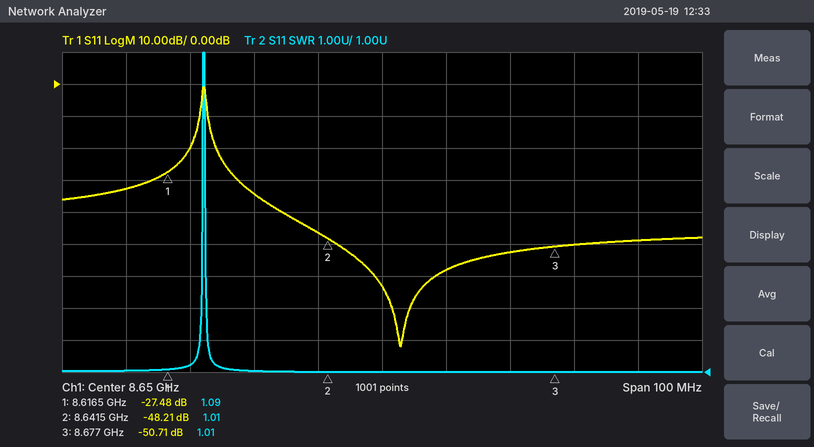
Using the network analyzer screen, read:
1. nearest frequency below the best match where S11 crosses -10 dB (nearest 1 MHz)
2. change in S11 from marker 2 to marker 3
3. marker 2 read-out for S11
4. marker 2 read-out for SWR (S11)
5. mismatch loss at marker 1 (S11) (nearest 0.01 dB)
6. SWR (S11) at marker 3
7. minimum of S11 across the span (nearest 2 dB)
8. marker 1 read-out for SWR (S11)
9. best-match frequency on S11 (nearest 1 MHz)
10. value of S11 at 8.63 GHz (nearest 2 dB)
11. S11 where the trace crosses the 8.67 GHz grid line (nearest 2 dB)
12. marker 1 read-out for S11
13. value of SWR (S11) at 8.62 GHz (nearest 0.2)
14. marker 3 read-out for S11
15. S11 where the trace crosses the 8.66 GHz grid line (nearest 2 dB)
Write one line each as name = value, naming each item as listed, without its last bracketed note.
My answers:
nearest frequency below the best match where S11 crosses -10 dB = 8.623 GHz
change in S11 from marker 2 to marker 3 = -2.50 dB
marker 2 read-out for S11 = -48.21 dB
marker 2 read-out for SWR = 1.01
mismatch loss at marker 1 (S11) = 0.01 dB
SWR (S11) at marker 3 = 1.01
minimum of S11 across the span = -82 dB
marker 1 read-out for SWR = 1.09
best-match frequency on S11 = 8.653 GHz
value of S11 at 8.63 GHz = -34 dB
S11 where the trace crosses the 8.67 GHz grid line = -52 dB
marker 1 read-out for S11 = -27.48 dB
value of SWR (S11) at 8.62 GHz = 1.2
marker 3 read-out for S11 = -50.71 dB
S11 where the trace crosses the 8.66 GHz grid line = -58 dB
